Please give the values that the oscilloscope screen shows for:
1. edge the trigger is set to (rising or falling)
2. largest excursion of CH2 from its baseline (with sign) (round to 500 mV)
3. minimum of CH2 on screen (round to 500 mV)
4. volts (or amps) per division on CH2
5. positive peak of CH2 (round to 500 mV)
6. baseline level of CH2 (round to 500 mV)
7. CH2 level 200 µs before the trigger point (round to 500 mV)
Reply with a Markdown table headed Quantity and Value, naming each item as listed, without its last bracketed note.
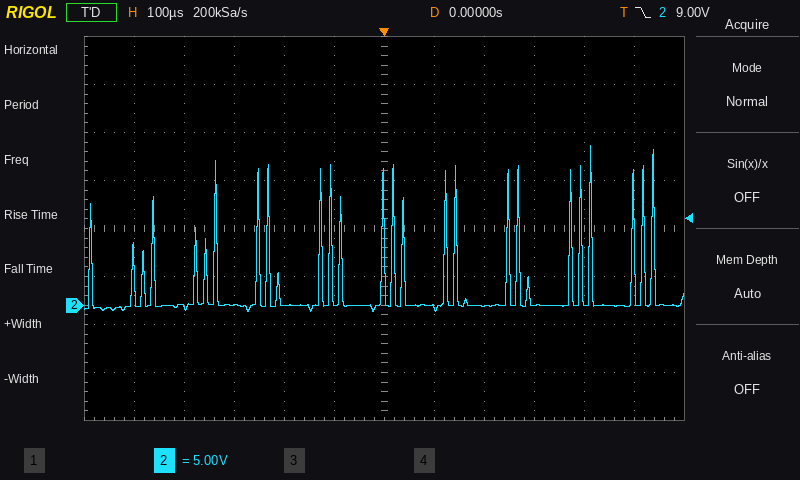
| Quantity | Value |
|---|---|
| edge the trigger is set to | falling |
| largest excursion of CH2 from its baseline (with sign) | +16.5 V |
| minimum of CH2 on screen | -500 mV |
| volts (or amps) per division on CH2 | 5 V |
| positive peak of CH2 | 16.5 V |
| baseline level of CH2 | 0.0 V |
| CH2 level 200 µs before the trigger point | 0.0 V |
